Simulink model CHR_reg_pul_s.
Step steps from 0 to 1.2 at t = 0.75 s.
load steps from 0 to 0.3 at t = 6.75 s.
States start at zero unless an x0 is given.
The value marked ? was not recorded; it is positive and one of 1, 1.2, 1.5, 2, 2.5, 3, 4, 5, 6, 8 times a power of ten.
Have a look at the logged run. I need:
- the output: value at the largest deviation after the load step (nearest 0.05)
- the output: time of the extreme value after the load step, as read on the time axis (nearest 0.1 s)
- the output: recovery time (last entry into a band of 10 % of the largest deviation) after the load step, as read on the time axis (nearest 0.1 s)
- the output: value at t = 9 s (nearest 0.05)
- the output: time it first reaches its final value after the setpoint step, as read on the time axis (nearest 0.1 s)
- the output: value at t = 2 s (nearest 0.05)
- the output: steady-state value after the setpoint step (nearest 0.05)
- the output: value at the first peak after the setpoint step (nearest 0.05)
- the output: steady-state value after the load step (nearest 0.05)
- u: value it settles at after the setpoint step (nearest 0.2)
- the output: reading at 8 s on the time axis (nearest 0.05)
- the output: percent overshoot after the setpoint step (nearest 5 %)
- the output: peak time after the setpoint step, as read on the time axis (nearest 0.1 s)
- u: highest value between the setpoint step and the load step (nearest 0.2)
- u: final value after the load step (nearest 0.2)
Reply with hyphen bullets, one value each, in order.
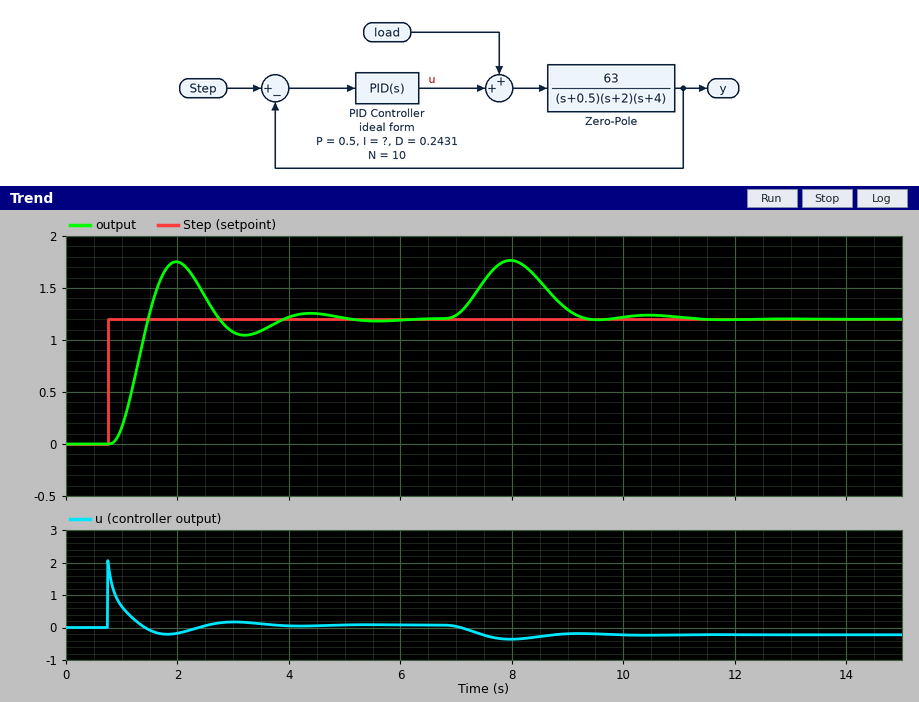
- 1.75
- 8.0 s
- 9.1 s
- 1.30
- 1.5 s
- 1.75
- 1.20
- 1.75
- 1.20
- 0.0
- 1.75
- 45 %
- 2.0 s
- 2.0
- -0.2
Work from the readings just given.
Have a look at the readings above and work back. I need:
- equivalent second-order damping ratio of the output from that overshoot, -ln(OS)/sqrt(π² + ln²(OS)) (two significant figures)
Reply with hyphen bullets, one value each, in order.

- 0.25
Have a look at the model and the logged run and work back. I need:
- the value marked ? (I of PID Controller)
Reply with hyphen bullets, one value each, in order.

- 0.8
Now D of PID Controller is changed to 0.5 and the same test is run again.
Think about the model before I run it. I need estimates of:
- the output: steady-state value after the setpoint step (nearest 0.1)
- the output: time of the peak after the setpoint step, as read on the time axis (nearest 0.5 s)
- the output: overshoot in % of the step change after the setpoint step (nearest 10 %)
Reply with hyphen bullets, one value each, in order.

- 1.2
- 1.5 s
- 30 %
